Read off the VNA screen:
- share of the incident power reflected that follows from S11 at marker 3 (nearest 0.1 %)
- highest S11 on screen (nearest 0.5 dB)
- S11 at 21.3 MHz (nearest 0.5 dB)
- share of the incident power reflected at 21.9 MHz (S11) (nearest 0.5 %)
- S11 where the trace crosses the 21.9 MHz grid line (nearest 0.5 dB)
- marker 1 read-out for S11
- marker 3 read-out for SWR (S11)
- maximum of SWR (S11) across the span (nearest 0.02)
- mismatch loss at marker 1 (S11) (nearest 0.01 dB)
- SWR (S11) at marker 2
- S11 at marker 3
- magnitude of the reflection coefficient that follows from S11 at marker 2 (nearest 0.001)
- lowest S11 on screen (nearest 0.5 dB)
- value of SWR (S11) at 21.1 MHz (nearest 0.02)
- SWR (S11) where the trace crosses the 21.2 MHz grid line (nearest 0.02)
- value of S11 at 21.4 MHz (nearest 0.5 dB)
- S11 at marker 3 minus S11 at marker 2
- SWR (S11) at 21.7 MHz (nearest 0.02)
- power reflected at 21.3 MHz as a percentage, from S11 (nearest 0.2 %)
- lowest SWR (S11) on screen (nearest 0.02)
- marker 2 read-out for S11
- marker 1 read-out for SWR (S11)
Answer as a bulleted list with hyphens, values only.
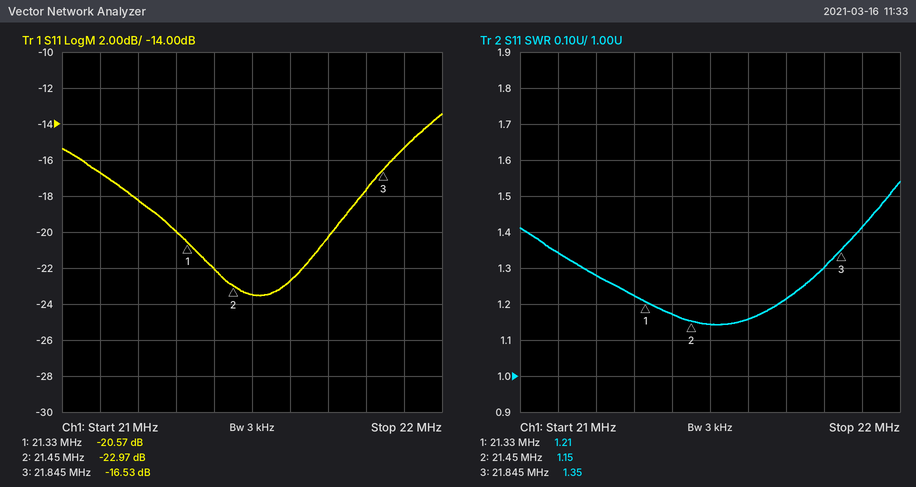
- 2.2 %
- -13.5 dB
- -20.0 dB
- 3.0 %
- -15.5 dB
- -20.57 dB
- 1.35
- 1.54
- 0.04 dB
- 1.15
- -16.53 dB
- 0.071
- -23.5 dB
- 1.34
- 1.28
- -22.0 dB
- 6.44 dB
- 1.22
- 1.0 %
- 1.14
- -22.97 dB
- 1.21
